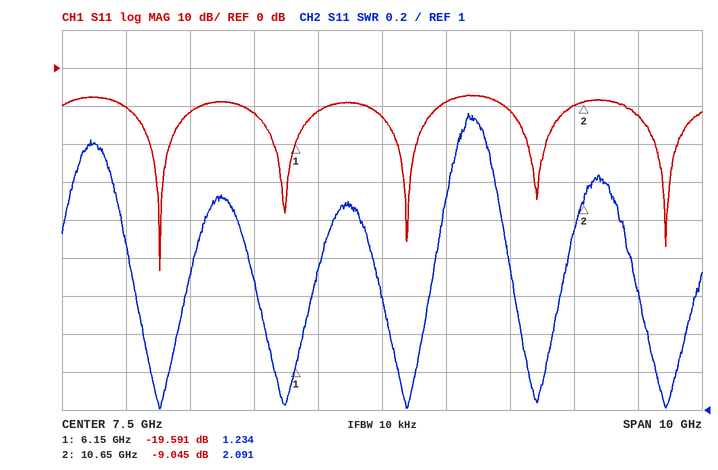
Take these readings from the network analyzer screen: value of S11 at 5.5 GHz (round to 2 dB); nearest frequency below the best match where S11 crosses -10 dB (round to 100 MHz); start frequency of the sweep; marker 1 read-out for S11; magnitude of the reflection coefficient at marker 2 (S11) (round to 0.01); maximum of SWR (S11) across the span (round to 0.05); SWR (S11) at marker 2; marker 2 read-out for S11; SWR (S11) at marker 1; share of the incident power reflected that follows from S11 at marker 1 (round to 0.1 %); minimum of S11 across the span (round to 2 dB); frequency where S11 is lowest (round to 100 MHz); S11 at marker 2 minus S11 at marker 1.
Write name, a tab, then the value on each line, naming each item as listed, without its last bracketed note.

value of S11 at 5.5 GHz	-12 dB
nearest frequency below the best match where S11 crosses -10 dB	3.5 GHz
start frequency of the sweep	2.5 GHz
marker 1 read-out for S11	-19.591 dB
magnitude of the reflection coefficient at marker 2 (S11)	0.35
maximum of SWR (S11) across the span	2.55
SWR (S11) at marker 2	2.091
marker 2 read-out for S11	-9.045 dB
SWR (S11) at marker 1	1.234
share of the incident power reflected that follows from S11 at marker 1	1.1 %
minimum of S11 across the span	-54 dB
frequency where S11 is lowest	4.0 GHz
S11 at marker 2 minus S11 at marker 1	10.546 dB
